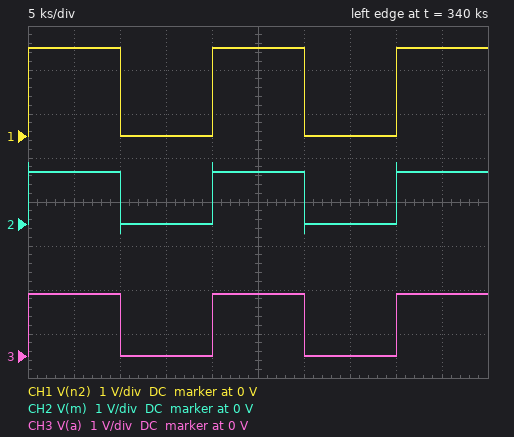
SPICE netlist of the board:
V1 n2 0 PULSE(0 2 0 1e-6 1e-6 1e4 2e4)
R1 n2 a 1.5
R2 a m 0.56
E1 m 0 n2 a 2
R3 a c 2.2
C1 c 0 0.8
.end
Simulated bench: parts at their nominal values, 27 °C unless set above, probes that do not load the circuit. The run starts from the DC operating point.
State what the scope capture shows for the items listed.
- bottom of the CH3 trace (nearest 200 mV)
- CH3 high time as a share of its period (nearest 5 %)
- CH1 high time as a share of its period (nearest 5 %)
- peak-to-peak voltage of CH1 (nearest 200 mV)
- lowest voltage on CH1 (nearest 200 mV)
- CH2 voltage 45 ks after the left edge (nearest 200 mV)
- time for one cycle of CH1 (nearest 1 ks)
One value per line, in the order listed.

0 V
50 %
50 %
2.0 V
0 V
1.2 V
20 ks
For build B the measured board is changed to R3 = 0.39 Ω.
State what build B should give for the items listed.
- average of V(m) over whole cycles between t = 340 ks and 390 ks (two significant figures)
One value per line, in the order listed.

590 mV
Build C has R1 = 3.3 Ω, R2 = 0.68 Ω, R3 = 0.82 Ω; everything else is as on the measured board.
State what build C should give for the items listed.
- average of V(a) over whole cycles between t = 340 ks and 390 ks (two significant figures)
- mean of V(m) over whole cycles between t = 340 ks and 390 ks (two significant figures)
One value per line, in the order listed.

690 mV
620 mV
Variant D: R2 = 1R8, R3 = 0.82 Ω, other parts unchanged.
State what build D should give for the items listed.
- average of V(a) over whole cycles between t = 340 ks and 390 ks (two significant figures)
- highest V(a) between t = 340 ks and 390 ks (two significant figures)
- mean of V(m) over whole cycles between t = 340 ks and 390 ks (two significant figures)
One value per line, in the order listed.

760 mV
1.5 V
480 mV
